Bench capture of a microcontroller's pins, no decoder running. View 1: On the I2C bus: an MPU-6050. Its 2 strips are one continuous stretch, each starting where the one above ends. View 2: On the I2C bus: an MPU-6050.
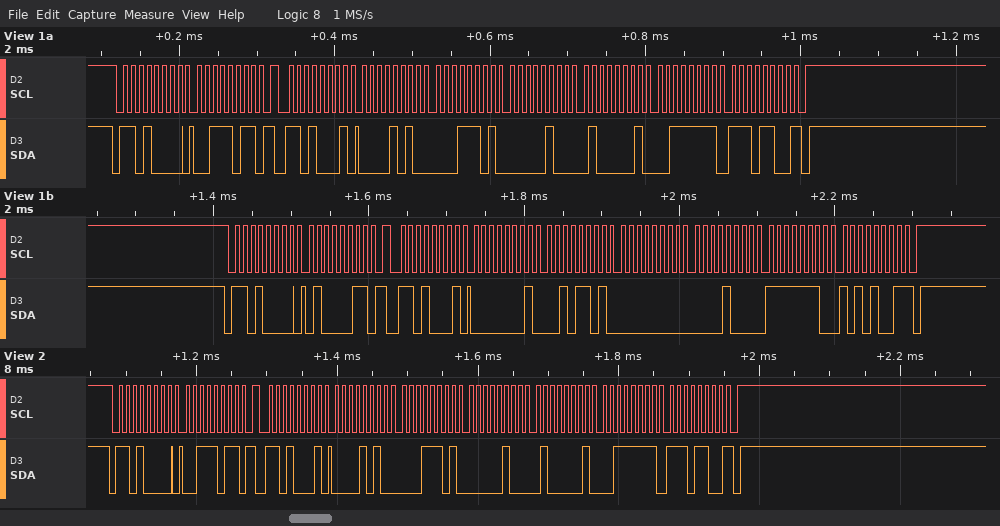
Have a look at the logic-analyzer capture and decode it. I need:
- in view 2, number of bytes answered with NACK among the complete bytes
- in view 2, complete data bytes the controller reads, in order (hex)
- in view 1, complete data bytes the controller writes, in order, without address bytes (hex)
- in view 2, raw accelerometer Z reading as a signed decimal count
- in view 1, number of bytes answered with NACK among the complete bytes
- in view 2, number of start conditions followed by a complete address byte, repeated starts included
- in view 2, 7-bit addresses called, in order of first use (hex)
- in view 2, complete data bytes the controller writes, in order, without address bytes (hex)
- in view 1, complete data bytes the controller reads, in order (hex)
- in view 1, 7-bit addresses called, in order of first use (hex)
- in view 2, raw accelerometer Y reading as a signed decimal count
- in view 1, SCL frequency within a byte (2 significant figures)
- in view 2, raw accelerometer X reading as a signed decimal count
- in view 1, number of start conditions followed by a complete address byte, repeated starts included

1
0A 1D 04 41 3F EC
3B 43
16364
2
2
0x68
3B
0A 1D 04 41 3F EC 01 2D 00 08 FE A9
0x68
1089
100 kHz
2589
4
